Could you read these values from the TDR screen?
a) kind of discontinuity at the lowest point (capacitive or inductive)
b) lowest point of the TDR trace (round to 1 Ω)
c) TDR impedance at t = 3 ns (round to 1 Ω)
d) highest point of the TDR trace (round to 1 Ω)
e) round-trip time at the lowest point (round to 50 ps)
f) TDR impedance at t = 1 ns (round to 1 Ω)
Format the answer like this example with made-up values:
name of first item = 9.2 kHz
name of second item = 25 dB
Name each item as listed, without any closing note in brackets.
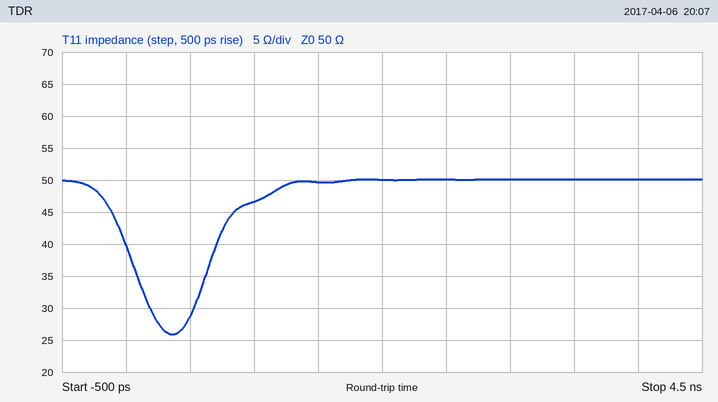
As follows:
kind of discontinuity at the lowest point = capacitive
lowest point of the TDR trace = 26 Ω
TDR impedance at t = 3 ns = 50 Ω
highest point of the TDR trace = 50 Ω
round-trip time at the lowest point = 350 ps
TDR impedance at t = 1 ns = 47 Ω
